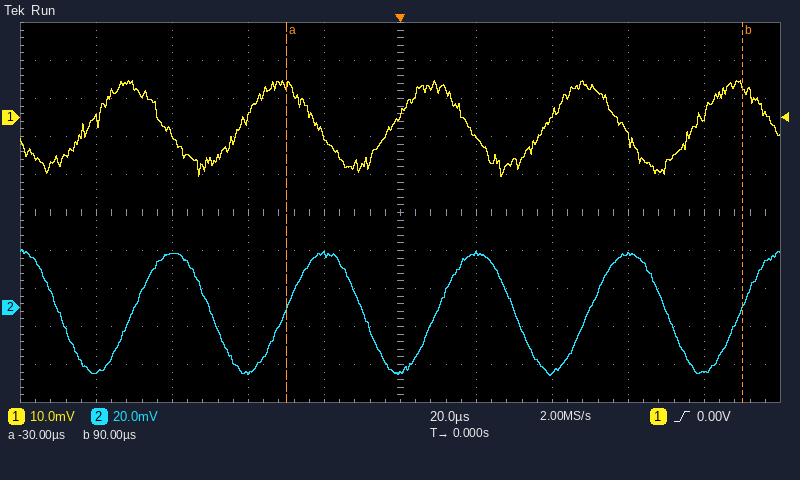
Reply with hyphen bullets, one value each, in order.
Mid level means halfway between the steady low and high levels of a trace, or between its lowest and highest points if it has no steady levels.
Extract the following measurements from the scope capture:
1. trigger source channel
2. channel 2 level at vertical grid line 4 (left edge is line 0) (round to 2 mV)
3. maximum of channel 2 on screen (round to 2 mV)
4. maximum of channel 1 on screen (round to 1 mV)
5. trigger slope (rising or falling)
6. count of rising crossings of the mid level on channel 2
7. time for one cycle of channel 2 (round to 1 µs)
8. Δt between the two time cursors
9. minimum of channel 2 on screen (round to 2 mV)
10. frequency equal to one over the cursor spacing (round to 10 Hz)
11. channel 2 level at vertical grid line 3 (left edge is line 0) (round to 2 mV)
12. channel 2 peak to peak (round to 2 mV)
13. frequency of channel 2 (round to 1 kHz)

- channel 1
- 28 mV
- 30 mV
- 10 mV
- rising
- 5
- 40 µs
- 120 µs
- -36 mV
- 8.33 kHz
- -34 mV
- 66 mV
- 25 kHz
